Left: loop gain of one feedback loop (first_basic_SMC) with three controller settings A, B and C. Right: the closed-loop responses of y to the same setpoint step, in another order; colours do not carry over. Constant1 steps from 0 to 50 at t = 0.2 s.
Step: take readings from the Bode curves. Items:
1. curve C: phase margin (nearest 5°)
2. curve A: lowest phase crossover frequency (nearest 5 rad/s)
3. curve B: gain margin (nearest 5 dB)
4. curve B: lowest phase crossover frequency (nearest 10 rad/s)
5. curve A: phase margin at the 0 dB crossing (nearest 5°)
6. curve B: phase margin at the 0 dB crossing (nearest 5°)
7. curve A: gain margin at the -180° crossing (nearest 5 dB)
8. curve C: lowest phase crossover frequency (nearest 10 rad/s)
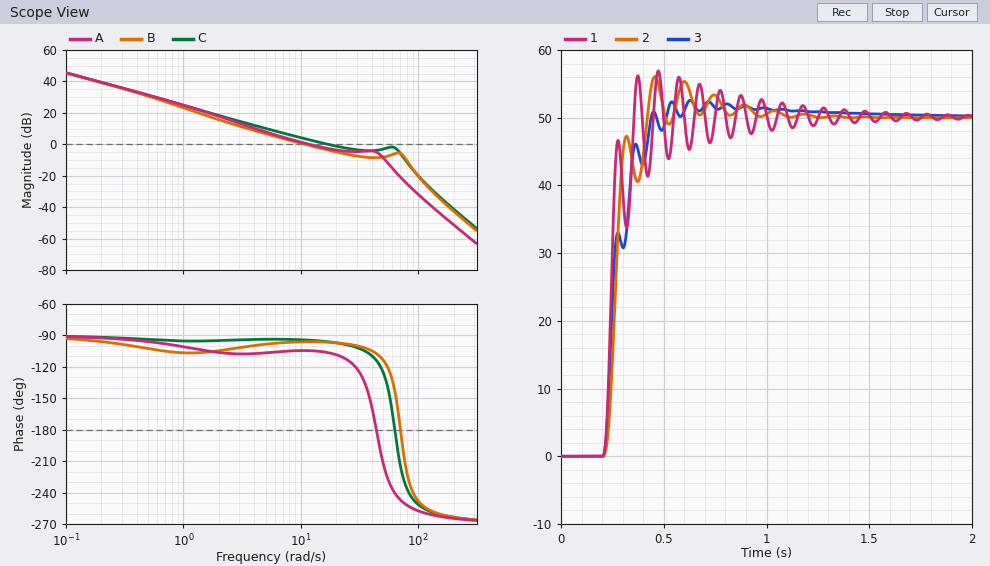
85°
45 rad/s
5 dB
70 rad/s
75°
85°
5 dB
60 rad/s
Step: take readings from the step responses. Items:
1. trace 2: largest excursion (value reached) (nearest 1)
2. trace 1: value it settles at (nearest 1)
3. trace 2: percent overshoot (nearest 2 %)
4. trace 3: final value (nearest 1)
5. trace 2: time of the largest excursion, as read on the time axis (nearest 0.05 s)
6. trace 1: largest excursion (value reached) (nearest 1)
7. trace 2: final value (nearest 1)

56
50
12 %
50
0.45 s
57
50
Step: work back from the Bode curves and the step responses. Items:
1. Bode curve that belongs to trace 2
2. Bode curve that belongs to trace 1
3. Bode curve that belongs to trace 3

A
C
B
